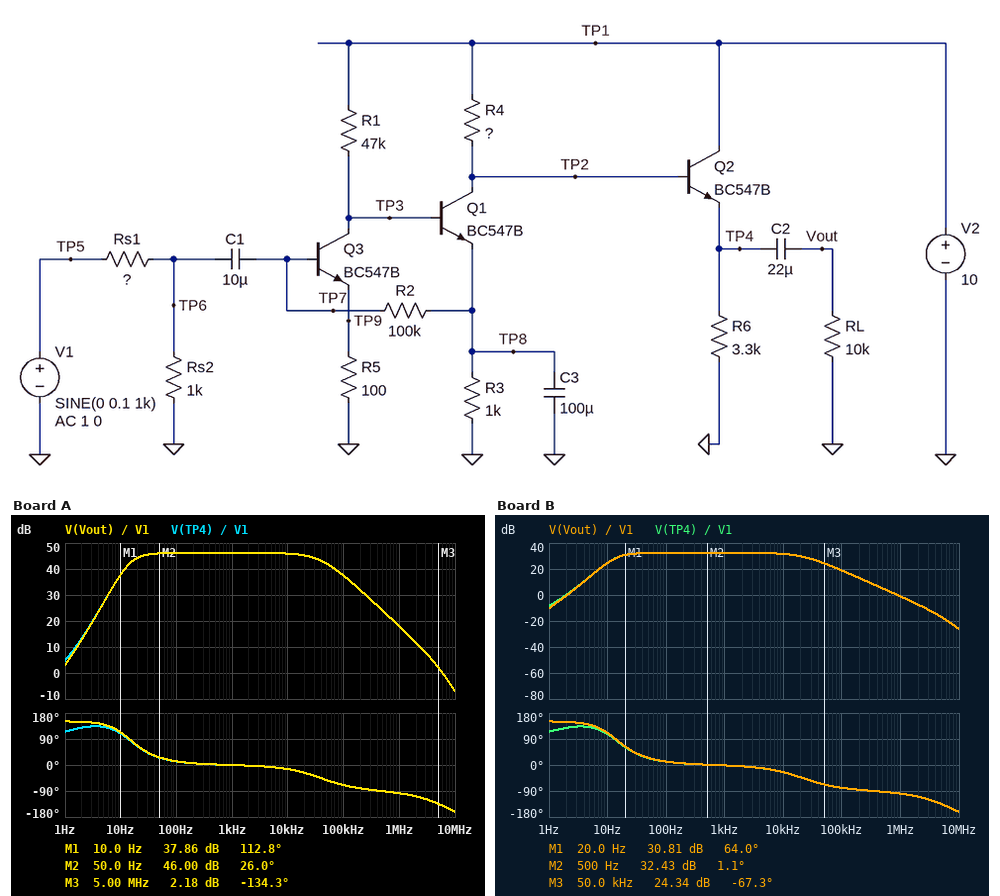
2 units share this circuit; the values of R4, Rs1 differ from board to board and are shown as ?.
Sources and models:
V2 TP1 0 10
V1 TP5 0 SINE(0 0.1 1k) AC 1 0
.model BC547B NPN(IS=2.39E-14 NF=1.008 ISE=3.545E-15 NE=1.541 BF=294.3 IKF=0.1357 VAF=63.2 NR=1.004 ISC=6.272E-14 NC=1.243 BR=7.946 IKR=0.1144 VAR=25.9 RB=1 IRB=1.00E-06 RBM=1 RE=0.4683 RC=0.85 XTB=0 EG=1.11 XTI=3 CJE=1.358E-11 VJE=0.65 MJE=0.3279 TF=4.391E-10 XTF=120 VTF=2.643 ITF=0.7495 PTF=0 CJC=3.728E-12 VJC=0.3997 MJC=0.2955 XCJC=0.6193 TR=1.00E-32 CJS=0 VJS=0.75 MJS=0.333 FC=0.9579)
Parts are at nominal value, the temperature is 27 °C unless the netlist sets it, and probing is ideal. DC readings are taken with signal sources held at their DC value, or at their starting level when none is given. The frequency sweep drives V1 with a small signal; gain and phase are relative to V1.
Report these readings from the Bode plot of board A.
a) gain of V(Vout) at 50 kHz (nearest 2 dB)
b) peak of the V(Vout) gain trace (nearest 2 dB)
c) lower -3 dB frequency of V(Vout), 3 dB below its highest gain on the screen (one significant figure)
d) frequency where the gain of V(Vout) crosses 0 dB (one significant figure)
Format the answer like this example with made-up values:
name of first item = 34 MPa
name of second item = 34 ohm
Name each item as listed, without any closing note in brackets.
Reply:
gain of V(Vout) at 50 kHz = 42 dB
peak of the V(Vout) gain trace = 46 dB
lower -3 dB frequency of V(Vout), 3 dB below its highest gain on the screen = 20 Hz
frequency where the gain of V(Vout) crosses 0 dB = 6 MHz
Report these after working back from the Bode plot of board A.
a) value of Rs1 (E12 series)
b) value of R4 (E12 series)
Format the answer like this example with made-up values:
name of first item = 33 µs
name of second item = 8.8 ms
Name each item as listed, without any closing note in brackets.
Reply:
value of Rs1 = 33 kΩ
value of R4 = 8.2 kΩ
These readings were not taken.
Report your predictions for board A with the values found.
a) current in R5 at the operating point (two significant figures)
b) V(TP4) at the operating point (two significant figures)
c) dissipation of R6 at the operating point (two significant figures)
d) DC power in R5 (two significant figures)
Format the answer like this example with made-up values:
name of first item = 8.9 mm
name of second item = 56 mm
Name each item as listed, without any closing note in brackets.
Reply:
current in R5 at the operating point = 180 µA
V(TP4) at the operating point = 3.8 V
dissipation of R6 at the operating point = 4.4 mW
DC power in R5 = 3.4 µW
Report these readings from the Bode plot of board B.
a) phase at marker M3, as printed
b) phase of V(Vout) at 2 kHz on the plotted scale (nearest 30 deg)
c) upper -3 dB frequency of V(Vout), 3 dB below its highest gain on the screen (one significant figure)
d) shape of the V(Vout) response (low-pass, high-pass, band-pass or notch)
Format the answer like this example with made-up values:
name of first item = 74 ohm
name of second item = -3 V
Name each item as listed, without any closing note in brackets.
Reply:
phase at marker M3, as printed = -67.3 deg
phase of V(Vout) at 2 kHz on the plotted scale = 0 deg
upper -3 dB frequency of V(Vout), 3 dB below its highest gain on the screen = 20 kHz
shape of the V(Vout) response = band-pass
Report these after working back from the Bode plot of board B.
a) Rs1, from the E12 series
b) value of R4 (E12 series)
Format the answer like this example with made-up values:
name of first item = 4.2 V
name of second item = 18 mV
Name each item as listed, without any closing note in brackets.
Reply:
Rs1, from the E12 series = 220 kΩ
value of R4 = 12 kΩ
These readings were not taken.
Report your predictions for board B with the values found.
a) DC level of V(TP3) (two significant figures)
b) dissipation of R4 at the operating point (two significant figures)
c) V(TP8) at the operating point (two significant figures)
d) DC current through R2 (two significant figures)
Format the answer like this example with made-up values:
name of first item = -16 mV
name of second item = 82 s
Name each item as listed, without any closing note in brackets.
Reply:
DC level of V(TP3) = 1.3 V
dissipation of R4 at the operating point = 5.5 mW
V(TP8) at the operating point = 680 mV
DC current through R2 = 640 nA
